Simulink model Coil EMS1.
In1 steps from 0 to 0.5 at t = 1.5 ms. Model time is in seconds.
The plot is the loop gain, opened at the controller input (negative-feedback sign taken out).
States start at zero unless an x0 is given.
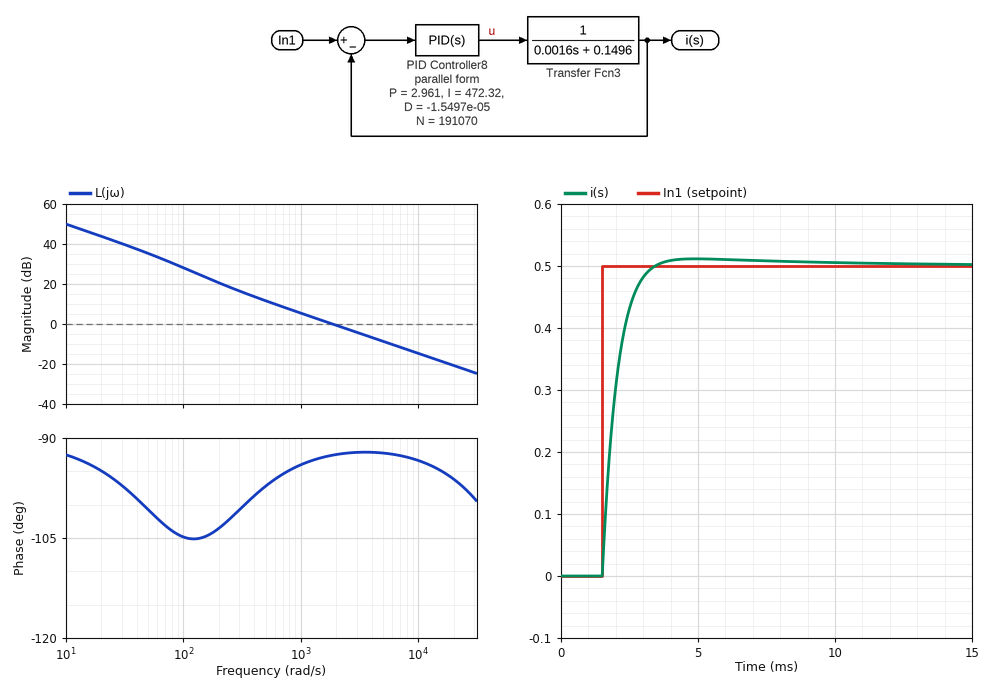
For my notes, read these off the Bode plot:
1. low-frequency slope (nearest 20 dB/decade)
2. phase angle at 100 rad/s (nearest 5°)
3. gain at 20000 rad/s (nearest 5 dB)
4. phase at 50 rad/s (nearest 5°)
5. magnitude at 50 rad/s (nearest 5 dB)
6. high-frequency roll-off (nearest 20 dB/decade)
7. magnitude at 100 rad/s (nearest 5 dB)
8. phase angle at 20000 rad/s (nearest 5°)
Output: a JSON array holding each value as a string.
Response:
["-20 dB/decade", "-105°", "-20 dB", "-100°", "35 dB", "-20 dB/decade", "30 dB", "-95°"]
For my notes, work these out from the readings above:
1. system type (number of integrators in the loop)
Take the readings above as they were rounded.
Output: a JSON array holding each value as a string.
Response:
["1"]
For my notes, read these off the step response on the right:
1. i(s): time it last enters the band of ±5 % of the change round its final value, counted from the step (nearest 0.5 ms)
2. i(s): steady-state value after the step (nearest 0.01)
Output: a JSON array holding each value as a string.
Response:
["1.5 ms", "0.50"]
